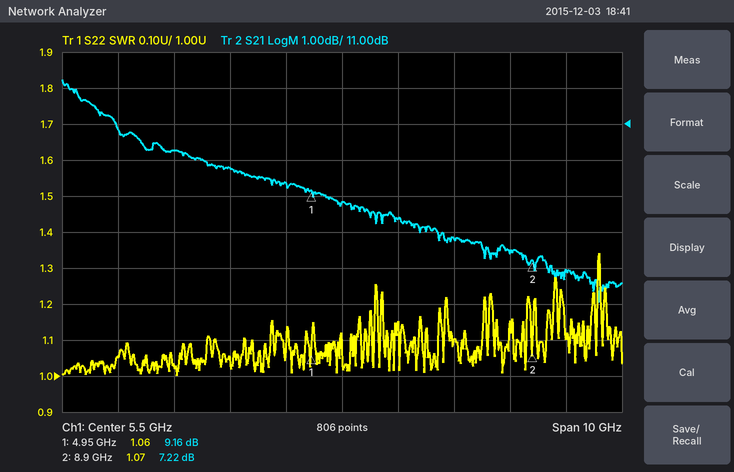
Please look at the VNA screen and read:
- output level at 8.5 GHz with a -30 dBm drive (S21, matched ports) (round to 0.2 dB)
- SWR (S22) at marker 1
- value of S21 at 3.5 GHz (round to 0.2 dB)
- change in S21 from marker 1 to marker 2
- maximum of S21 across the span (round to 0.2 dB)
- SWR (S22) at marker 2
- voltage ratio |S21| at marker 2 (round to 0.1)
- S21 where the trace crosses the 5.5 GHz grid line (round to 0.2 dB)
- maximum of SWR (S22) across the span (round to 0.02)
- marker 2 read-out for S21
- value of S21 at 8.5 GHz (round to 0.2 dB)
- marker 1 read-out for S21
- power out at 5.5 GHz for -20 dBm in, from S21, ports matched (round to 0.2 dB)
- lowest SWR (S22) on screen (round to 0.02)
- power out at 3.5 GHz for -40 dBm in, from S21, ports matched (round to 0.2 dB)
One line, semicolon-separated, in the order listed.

-22.6 dBm; 1.06; 9.8 dB; -1.94 dB; 12.2 dB; 1.07; 2.3; 8.8 dB; 1.34; 7.22 dB; 7.4 dB; 9.16 dB; -11.2 dBm; 1.00; -30.2 dBm
